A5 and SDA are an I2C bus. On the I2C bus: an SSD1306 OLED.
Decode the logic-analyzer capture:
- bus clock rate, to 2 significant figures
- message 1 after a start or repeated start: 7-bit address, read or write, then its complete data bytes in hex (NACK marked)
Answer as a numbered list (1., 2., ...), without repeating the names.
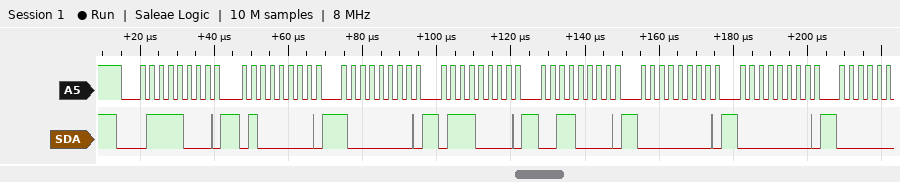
1. 400 kHz
2. 0x3C write: 40 80 70 30 00 00
